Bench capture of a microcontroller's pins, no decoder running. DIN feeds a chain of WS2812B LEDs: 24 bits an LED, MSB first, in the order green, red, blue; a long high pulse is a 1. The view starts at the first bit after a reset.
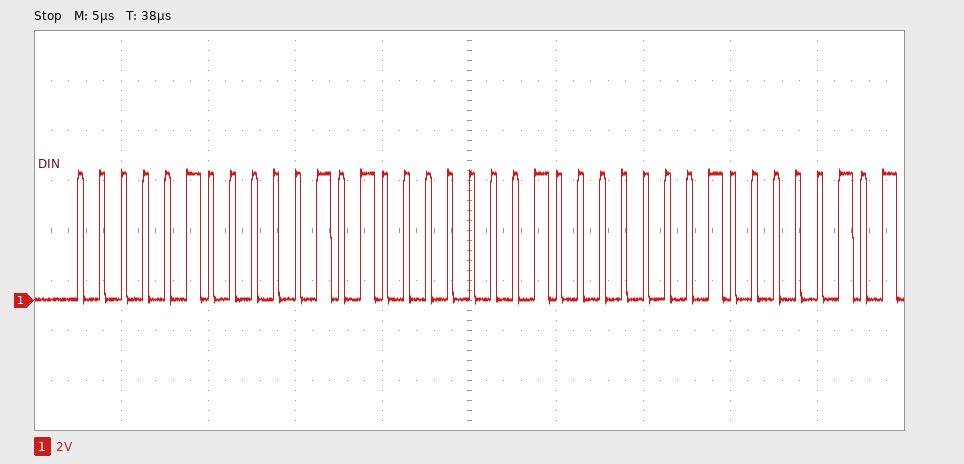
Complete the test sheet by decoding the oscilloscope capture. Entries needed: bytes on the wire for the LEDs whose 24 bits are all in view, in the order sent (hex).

04 14 04
